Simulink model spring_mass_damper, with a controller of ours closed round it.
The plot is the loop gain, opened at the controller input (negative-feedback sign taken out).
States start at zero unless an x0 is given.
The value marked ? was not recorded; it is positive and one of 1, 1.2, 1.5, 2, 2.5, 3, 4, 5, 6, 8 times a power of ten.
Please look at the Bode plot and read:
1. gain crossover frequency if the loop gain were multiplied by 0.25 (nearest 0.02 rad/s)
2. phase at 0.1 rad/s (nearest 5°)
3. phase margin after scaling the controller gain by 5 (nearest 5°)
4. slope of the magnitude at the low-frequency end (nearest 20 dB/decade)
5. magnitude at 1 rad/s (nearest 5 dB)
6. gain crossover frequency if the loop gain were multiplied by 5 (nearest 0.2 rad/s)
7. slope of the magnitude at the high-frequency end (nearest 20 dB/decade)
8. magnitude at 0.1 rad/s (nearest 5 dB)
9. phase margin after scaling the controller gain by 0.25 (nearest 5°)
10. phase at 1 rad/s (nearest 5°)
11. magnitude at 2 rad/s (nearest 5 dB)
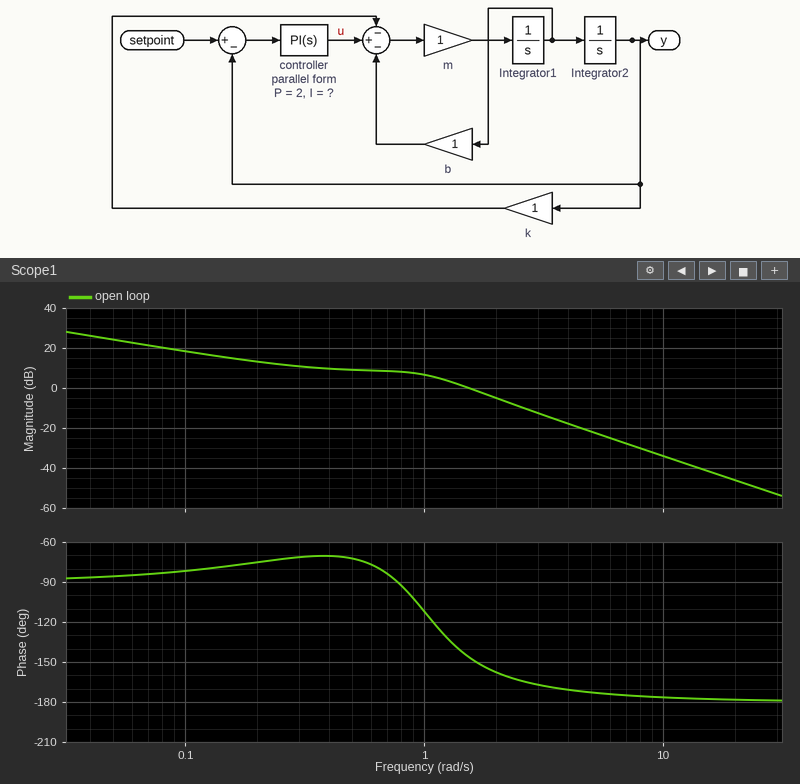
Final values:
0.24 rad/s
-80°
10°
-20 dB/decade
5 dB
3.2 rad/s
-40 dB/decade
20 dB
105°
-110°
-5 dB
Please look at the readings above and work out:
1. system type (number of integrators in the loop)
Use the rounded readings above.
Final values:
1
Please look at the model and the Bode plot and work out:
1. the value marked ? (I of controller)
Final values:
0.8
